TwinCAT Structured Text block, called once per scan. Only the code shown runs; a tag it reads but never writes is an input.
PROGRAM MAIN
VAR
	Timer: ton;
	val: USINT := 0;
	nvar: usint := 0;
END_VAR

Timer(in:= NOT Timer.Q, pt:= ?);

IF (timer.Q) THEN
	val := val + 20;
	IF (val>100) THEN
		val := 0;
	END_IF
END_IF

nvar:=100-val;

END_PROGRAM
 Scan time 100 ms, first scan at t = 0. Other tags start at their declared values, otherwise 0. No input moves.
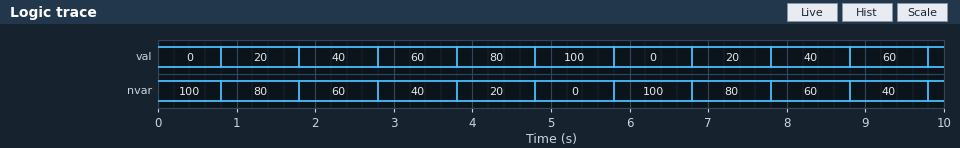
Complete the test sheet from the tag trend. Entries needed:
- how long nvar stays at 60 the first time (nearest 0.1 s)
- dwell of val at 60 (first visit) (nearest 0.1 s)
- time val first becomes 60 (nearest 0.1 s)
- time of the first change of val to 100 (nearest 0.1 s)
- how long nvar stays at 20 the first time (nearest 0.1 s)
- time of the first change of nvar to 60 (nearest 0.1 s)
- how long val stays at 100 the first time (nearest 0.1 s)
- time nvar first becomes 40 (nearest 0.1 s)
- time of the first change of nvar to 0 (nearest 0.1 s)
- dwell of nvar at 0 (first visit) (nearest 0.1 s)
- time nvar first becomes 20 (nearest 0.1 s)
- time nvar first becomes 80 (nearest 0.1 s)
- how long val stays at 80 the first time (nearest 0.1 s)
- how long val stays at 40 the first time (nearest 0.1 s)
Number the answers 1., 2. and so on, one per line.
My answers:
1. 1.0 s
2. 1.0 s
3. 2.8 s
4. 4.8 s
5. 1.0 s
6. 1.8 s
7. 1.0 s
8. 2.8 s
9. 4.8 s
10. 1.0 s
11. 3.8 s
12. 0.8 s
13. 1.0 s
14. 1.0 s
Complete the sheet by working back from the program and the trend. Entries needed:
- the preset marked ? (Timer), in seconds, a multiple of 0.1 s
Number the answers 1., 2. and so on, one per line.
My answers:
1. 0.8 s
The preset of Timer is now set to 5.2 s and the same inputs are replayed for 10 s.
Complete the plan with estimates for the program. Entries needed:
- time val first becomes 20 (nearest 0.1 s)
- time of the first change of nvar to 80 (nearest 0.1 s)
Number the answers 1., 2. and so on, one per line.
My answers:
1. 5.2 s
2. 5.2 s
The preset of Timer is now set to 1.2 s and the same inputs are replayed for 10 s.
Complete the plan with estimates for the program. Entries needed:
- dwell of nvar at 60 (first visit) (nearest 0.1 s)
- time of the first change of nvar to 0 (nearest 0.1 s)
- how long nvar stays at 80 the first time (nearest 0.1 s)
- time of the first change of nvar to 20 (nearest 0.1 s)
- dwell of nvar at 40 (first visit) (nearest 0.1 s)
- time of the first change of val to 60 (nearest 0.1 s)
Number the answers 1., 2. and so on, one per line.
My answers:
1. 1.4 s
2. 6.8 s
3. 1.4 s
4. 5.4 s
5. 1.4 s
6. 4.0 s
